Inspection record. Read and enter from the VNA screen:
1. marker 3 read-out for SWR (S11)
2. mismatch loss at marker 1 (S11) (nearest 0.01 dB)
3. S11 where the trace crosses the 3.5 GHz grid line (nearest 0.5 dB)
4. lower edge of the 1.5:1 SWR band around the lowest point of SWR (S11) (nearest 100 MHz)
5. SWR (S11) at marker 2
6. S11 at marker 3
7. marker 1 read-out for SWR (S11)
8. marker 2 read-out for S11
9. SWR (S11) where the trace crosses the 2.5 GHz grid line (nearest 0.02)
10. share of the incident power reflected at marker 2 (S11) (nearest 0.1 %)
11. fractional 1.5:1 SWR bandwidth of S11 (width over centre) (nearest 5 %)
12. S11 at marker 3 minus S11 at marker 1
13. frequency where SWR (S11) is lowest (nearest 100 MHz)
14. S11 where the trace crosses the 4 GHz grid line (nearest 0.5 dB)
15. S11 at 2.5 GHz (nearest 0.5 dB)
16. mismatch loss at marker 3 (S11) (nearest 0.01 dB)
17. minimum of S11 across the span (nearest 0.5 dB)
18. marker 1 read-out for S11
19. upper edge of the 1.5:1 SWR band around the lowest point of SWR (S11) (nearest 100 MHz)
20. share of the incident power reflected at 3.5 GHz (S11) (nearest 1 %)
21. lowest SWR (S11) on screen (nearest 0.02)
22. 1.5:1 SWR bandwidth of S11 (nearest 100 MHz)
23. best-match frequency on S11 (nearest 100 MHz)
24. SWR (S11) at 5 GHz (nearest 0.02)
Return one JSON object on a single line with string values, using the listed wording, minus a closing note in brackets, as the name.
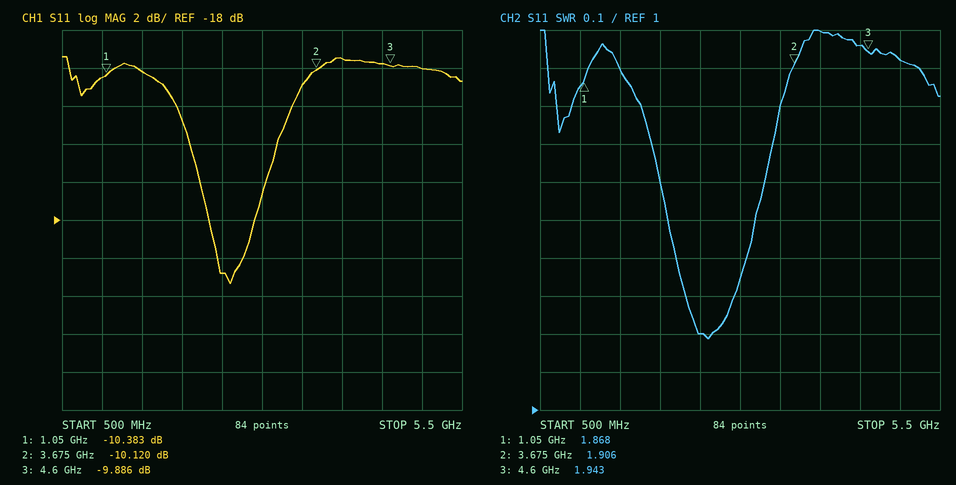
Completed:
{"marker 3 read-out for SWR": "1.943", "mismatch loss at marker 1 (S11)": "0.42 dB", "S11 where the trace crosses the 3.5 GHz grid line": "-11.0 dB", "lower edge of the 1.5:1 SWR band around the lowest point of SWR (S11)": "2.1 GHz", "SWR (S11) at marker 2": "1.906", "S11 at marker 3": "-9.886 dB", "marker 1 read-out for SWR": "1.868", "marker 2 read-out for S11": "-10.120 dB", "SWR (S11) where the trace crosses the 2.5 GHz grid line": "1.20", "share of the incident power reflected at marker 2 (S11)": "9.7 %", "fractional 1.5:1 SWR bandwidth of S11 (width over centre)": "40 %", "S11 at marker 3 minus S11 at marker 1": "0.497 dB", "frequency where SWR (S11) is lowest": "2.6 GHz", "S11 where the trace crosses the 4 GHz grid line": "-9.5 dB", "S11 at 2.5 GHz": "-21.0 dB", "mismatch loss at marker 3 (S11)": "0.47 dB", "minimum of S11 across the span": "-21.5 dB", "marker 1 read-out for S11": "-10.383 dB", "upper edge of the 1.5:1 SWR band around the lowest point of SWR (S11)": "3.2 GHz", "share of the incident power reflected at 3.5 GHz (S11)": "8 %", "lowest SWR (S11) on screen": "1.18", "1.5:1 SWR bandwidth of S11": "1.1 GHz", "best-match frequency on S11": "2.6 GHz", "SWR (S11) at 5 GHz": "1.92"}
